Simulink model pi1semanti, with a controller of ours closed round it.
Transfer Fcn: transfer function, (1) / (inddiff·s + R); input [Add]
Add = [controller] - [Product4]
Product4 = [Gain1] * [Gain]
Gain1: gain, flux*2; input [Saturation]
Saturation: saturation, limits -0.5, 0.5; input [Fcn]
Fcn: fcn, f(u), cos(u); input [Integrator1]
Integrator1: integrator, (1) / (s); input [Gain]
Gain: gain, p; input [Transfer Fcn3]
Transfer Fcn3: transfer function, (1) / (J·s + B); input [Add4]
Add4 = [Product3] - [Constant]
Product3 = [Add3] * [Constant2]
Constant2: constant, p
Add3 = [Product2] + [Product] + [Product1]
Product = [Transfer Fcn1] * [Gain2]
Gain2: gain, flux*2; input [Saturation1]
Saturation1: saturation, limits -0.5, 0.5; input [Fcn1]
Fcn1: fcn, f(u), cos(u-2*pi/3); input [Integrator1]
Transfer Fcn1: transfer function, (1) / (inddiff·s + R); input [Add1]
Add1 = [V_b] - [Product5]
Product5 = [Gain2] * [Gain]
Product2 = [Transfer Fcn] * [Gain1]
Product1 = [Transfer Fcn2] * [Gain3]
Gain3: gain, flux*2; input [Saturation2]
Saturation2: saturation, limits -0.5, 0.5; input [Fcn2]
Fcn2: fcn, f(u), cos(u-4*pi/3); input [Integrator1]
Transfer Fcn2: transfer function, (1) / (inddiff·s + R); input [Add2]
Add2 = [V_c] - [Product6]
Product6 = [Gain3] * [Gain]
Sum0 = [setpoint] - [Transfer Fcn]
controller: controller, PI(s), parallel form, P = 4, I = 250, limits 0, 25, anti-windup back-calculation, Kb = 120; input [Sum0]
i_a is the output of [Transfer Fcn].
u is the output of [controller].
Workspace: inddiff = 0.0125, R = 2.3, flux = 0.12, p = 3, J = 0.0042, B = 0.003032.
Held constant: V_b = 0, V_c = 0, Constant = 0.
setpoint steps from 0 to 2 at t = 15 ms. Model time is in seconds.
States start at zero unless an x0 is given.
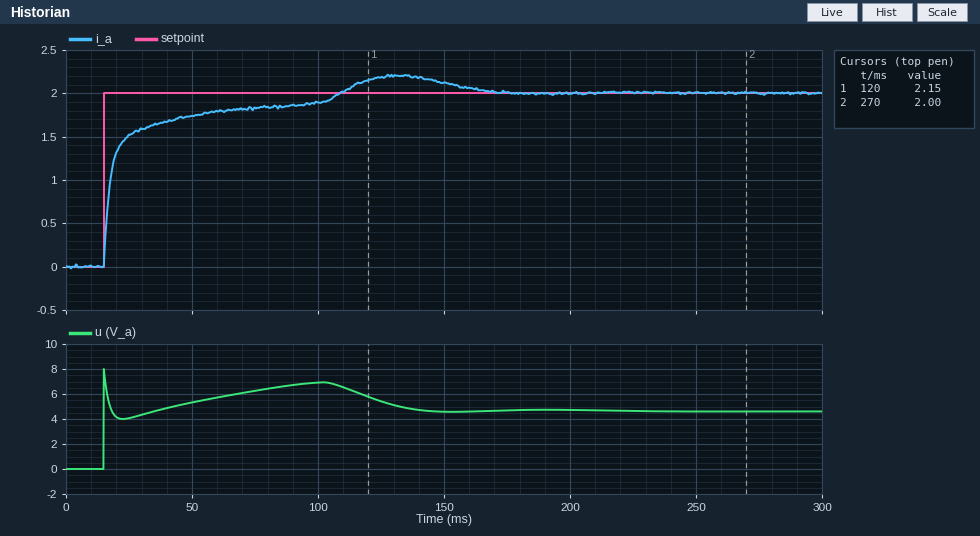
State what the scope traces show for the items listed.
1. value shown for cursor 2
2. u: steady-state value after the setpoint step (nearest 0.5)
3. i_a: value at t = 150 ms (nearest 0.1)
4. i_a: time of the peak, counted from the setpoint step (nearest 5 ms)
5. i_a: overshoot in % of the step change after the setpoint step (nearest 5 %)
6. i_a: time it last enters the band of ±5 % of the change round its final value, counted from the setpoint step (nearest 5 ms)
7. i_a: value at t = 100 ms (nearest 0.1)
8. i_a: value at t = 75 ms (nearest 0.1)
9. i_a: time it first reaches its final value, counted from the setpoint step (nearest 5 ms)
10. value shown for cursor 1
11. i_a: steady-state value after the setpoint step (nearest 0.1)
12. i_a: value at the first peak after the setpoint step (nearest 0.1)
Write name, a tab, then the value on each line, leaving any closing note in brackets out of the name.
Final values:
value shown for cursor 2	2.00
u: steady-state value after the setpoint step	4.5
i_a: value at t = 150 ms	2.1
i_a: time of the peak, counted from the setpoint step	115 ms
i_a: overshoot in % of the step change after the setpoint step	10 %
i_a: time it last enters the band of ±5 % of the change round its final value, counted from the setpoint step	140 ms
i_a: value at t = 100 ms	1.9
i_a: value at t = 75 ms	1.8
i_a: time it first reaches its final value, counted from the setpoint step	95 ms
value shown for cursor 1	2.15
i_a: steady-state value after the setpoint step	2.0
i_a: value at the first peak after the setpoint step	2.2
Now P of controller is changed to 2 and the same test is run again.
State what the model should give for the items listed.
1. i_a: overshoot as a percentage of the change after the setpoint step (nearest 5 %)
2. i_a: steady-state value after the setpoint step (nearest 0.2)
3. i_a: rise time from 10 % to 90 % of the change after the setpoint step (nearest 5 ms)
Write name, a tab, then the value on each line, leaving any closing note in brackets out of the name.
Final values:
i_a: overshoot as a percentage of the change after the setpoint step	15 %
i_a: steady-state value after the setpoint step	2.0
i_a: rise time from 10 % to 90 % of the change after the setpoint step	35 ms
